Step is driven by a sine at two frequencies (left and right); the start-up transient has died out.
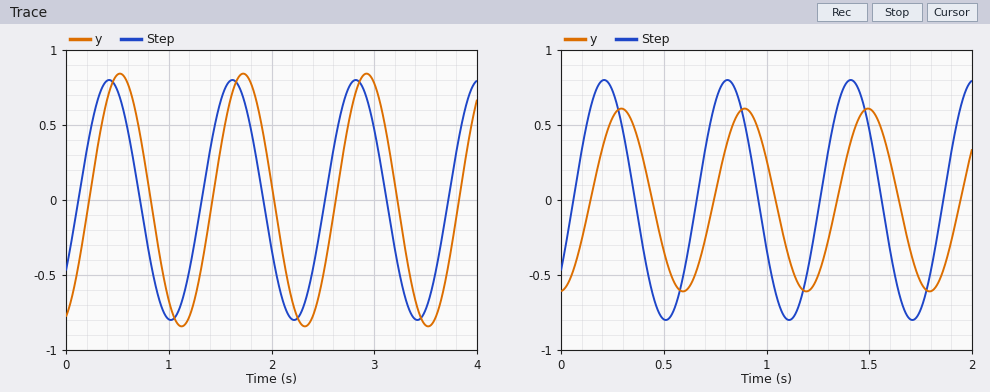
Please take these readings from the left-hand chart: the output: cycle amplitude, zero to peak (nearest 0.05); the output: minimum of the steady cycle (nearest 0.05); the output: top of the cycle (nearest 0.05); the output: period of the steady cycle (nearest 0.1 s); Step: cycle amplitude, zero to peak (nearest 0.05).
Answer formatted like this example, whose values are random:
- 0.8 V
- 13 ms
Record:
- 0.85
- -0.85
- 0.85
- 1.2 s
- 0.80
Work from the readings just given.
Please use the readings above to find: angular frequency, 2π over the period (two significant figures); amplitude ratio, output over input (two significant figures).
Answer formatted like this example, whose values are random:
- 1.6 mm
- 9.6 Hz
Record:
- 5.2 rad/s
- 1.1
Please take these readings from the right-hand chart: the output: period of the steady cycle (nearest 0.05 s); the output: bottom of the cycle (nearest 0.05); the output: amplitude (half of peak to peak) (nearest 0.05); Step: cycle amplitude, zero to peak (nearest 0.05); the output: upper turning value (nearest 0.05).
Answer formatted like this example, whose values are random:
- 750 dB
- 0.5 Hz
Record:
- 0.60 s
- -0.60
- 0.60
- 0.80
- 0.60
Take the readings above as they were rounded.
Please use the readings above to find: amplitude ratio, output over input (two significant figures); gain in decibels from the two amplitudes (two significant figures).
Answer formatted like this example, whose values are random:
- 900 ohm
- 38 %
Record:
- 0.75
- -2.5 dB
